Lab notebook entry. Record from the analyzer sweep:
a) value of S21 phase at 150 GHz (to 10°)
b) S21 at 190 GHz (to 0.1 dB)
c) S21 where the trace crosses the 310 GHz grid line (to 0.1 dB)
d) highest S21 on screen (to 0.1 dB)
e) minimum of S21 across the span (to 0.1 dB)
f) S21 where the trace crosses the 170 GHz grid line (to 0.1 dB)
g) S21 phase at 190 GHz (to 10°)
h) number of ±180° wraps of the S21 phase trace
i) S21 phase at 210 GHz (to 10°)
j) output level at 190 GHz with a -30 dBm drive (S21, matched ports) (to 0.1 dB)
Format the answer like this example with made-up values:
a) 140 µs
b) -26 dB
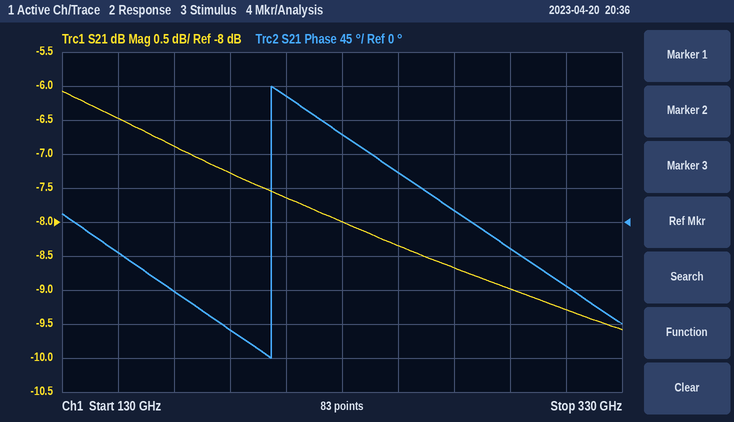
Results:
a) -40°
b) -7.3 dB
c) -9.3 dB
d) -6.1 dB
e) -9.6 dB
f) -6.9 dB
g) -140°
h) 1
i) 170°
j) -37.3 dBm
